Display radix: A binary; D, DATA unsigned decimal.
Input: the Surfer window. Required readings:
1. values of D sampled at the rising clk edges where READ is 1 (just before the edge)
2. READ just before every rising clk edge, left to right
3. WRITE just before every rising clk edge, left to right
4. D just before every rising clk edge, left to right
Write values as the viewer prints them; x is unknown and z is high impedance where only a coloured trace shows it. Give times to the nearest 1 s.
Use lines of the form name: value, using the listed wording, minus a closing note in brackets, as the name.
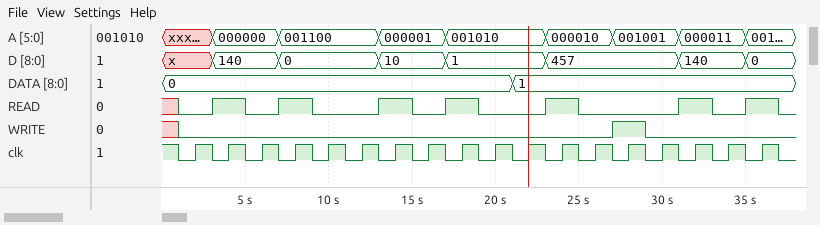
values of D sampled at the rising clk edges where READ is 1: 140, 0, 10, 1, 457, 140, 0
READ just before every rising clk edge, left to right: 0 1 0 1 0 0 1 0 1 0 0 1 0 0 0 1 0 1
WRITE just before every rising clk edge, left to right: 0 0 0 0 0 0 0 0 0 0 0 0 0 1 0 0 0 0
D just before every rising clk edge, left to right: x, 140, 140, 0, 0, 0, 10, 10, 1, 1, 1, 457, 457, 457, 457, 140, 140, 0
